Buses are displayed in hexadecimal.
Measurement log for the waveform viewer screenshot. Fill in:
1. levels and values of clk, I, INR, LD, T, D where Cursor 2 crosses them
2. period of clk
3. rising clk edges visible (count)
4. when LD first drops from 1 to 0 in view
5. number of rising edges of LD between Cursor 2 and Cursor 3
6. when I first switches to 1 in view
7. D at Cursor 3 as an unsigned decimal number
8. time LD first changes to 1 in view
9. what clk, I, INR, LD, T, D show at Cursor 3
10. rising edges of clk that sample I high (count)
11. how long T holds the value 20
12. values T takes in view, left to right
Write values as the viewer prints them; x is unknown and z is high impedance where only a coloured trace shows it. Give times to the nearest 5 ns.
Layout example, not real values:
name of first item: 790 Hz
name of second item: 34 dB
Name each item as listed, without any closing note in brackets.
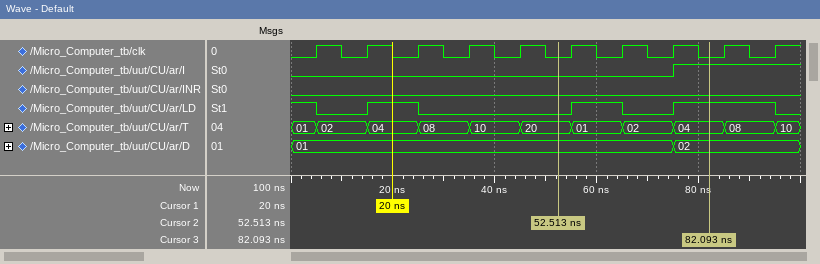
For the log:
levels and values of clk, I, INR, LD, T, D where Cursor 2 crosses them: clk=0, I=0, INR=0, LD=0, T=20, D=01
period of clk: 10 ns
rising clk edges visible: 10
when LD first drops from 1 to 0 in view: 5 ns
number of rising edges of LD between Cursor 2 and Cursor 3: 2
when I first switches to 1 in view: 75 ns
D at Cursor 3 as an unsigned decimal number: 2
time LD first changes to 1 in view: 15 ns
what clk, I, INR, LD, T, D show at Cursor 3: clk=0, I=1, INR=0, LD=1, T=04, D=02
rising edges of clk that sample I high: 2
how long T holds the value 20: 10 ns
values T takes in view, left to right: 01, 02, 04, 08, 10, 20, 01, 02, 04, 08, 10
